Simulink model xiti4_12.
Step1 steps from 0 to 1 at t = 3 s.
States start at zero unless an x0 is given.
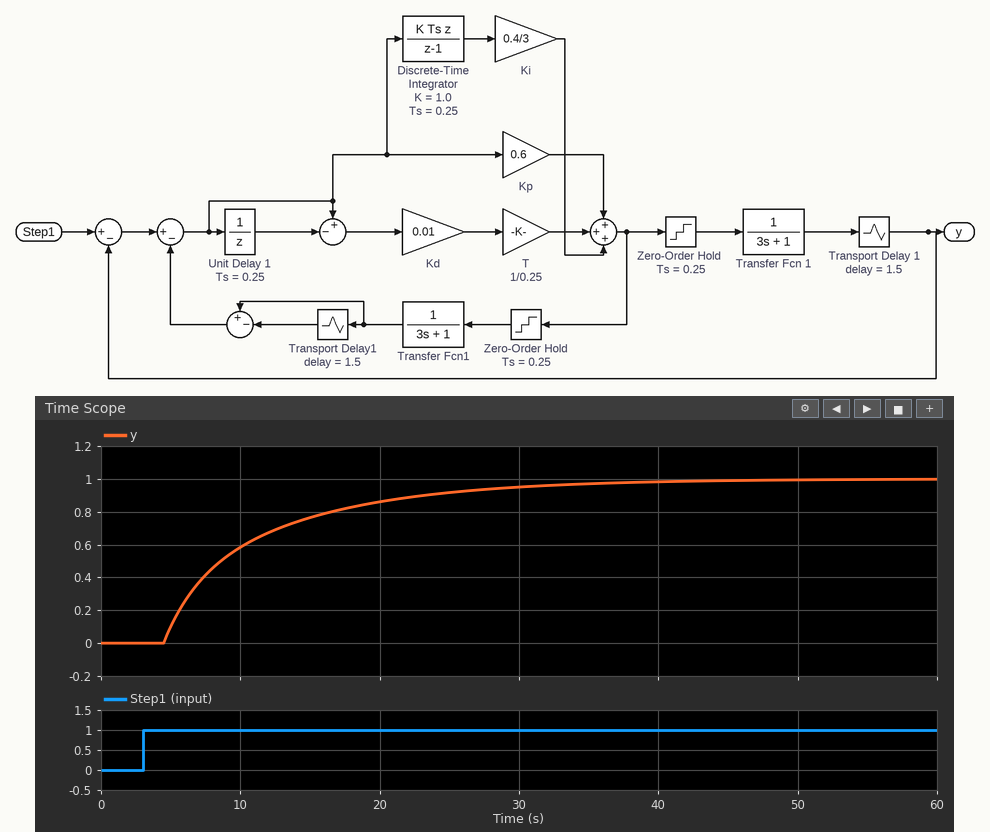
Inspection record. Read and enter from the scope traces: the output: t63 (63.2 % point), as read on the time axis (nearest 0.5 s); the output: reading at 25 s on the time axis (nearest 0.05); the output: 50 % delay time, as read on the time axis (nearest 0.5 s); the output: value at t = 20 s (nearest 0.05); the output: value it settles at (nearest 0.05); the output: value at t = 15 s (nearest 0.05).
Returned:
11.0 s
0.90
8.5 s
0.85
1.00
0.75
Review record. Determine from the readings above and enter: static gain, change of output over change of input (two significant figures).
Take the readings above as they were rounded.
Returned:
1.0
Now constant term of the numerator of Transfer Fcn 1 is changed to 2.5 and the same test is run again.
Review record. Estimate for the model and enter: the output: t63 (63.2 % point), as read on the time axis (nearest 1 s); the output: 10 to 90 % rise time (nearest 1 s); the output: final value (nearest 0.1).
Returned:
6 s
3 s
1.0
